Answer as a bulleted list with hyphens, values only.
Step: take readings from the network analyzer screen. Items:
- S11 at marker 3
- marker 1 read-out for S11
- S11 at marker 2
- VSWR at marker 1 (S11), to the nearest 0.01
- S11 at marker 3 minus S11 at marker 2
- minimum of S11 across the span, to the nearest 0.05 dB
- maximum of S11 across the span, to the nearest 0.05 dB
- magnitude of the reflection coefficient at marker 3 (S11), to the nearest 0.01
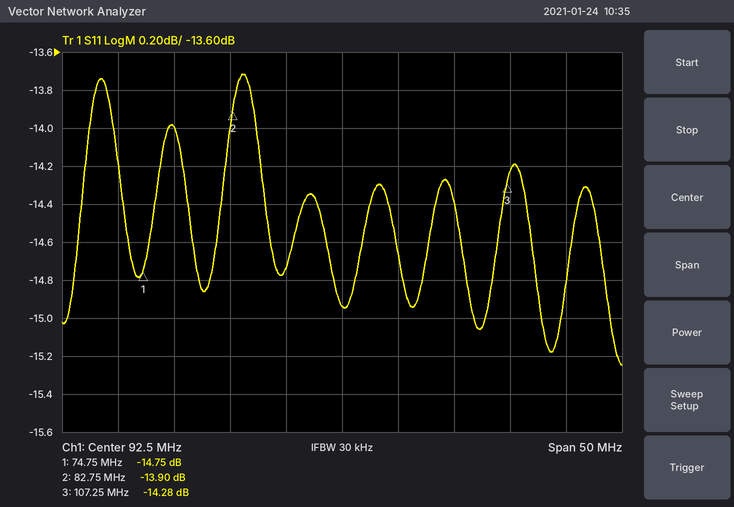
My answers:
- -14.28 dB
- -14.75 dB
- -13.90 dB
- 1.45
- -0.38 dB
- -15.25 dB
- -13.70 dB
- 0.19
